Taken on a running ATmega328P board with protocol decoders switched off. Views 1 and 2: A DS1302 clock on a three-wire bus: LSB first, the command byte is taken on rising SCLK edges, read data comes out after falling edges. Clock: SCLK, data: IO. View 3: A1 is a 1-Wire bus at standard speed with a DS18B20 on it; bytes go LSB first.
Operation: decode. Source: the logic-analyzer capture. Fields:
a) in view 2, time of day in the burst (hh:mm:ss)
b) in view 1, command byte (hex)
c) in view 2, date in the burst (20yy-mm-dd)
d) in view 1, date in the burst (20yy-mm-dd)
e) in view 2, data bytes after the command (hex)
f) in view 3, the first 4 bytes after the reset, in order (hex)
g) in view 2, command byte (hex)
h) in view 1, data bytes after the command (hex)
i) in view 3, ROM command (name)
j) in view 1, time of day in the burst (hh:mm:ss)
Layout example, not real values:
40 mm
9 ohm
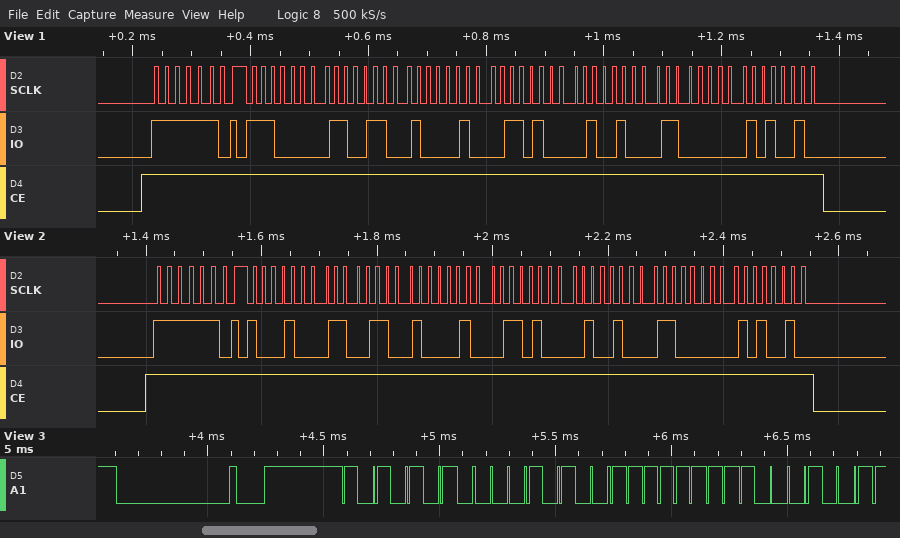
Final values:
21:33:11
0xBF
2025-12-16
2025-12-16
11 33 21 16 12 03 25
55 28 FF 91
0xBF
07 33 21 16 12 03 25
Match ROM
21:33:07
